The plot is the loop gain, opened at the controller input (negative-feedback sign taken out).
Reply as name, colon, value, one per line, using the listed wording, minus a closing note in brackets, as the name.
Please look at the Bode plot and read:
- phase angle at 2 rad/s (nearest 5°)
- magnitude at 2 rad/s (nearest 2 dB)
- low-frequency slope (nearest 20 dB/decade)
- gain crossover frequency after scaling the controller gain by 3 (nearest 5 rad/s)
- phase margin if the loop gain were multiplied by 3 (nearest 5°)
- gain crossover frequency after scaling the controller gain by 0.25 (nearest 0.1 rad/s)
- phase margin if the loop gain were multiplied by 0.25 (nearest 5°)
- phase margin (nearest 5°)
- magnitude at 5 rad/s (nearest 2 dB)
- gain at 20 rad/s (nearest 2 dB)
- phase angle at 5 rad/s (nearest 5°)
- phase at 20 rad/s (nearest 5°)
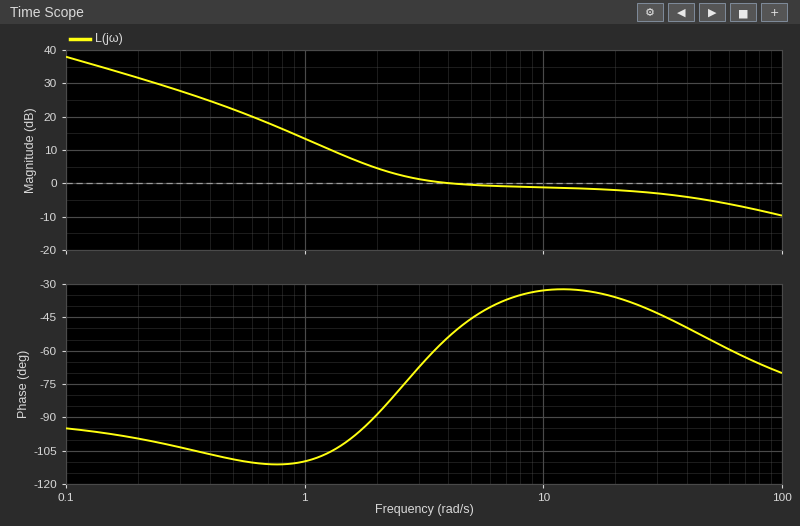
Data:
phase angle at 2 rad/s: -90°
magnitude at 2 rad/s: 4 dB
low-frequency slope: -20 dB/decade
gain crossover frequency after scaling the controller gain by 3: 100 rad/s
phase margin if the loop gain were multiplied by 3: 110°
gain crossover frequency after scaling the controller gain by 0.25: 1.1 rad/s
phase margin if the loop gain were multiplied by 0.25: 70°
phase margin: 125°
magnitude at 5 rad/s: 0 dB
gain at 20 rad/s: -2 dB
phase angle at 5 rad/s: -45°
phase at 20 rad/s: -35°
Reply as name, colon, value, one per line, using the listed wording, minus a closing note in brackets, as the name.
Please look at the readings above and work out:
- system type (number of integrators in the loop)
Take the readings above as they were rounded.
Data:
system type: 1
